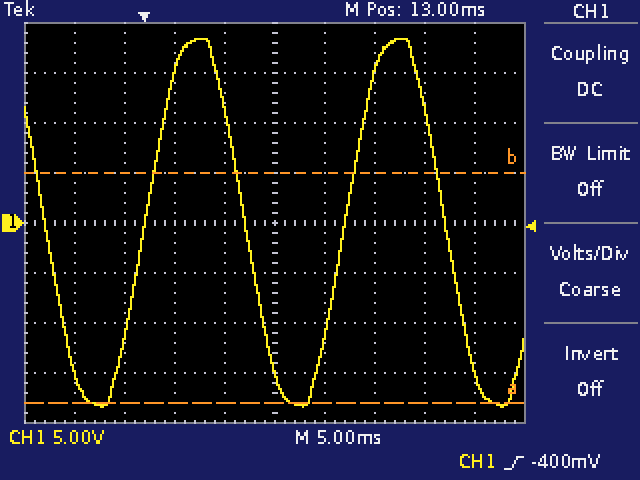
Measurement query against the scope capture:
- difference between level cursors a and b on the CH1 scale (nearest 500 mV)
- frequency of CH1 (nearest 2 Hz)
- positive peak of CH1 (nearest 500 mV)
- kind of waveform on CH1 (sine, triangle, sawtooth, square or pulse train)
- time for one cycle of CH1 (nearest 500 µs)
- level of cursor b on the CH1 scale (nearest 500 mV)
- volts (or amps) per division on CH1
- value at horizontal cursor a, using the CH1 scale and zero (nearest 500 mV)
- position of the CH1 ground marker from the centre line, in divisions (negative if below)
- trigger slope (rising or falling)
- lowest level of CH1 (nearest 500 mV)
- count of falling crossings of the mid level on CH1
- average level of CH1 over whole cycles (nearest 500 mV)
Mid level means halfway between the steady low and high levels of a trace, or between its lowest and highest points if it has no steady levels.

23.0 V
50 Hz
18.5 V
sine
20.0 ms
5.0 V
5 V
-18.0 V
0.0 div
rising
-18.5 V
3
0.0 V
